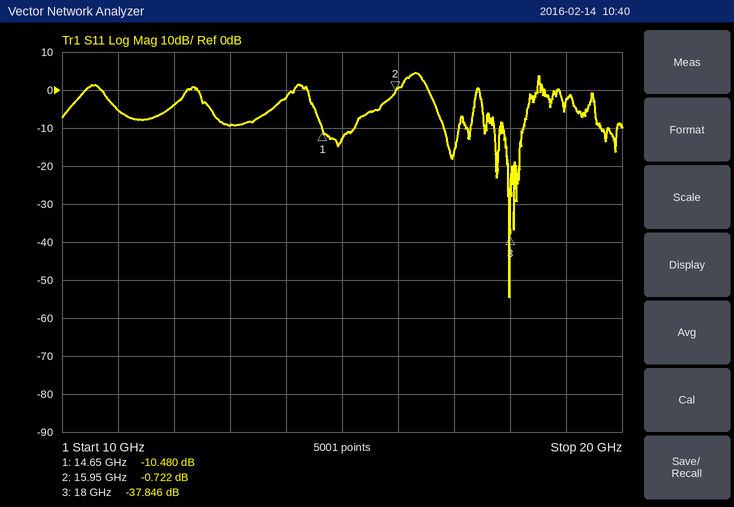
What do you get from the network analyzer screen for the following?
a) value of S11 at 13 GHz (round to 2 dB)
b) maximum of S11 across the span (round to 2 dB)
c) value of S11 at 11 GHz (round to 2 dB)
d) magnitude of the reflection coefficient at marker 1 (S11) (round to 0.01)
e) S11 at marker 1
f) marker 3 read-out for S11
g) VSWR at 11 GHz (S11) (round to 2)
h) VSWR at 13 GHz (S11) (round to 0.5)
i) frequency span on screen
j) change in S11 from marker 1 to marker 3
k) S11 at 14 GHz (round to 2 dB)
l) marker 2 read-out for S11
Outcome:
-10 dB
4 dB
-6 dB
0.30
-10.480 dB
-37.846 dB
4
2.0
10 GHz
-27.366 dB
-2 dB
-0.722 dB
